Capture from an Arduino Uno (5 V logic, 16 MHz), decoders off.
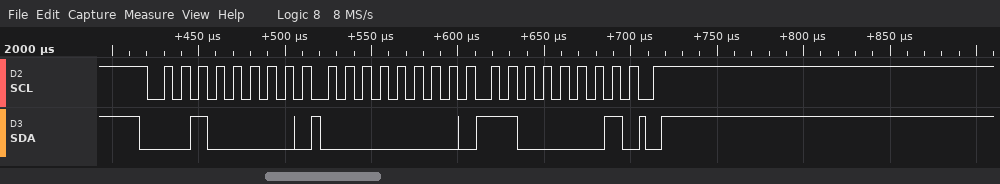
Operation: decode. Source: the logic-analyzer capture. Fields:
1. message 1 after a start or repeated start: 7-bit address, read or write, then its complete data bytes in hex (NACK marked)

0x10 write: 00 C1
